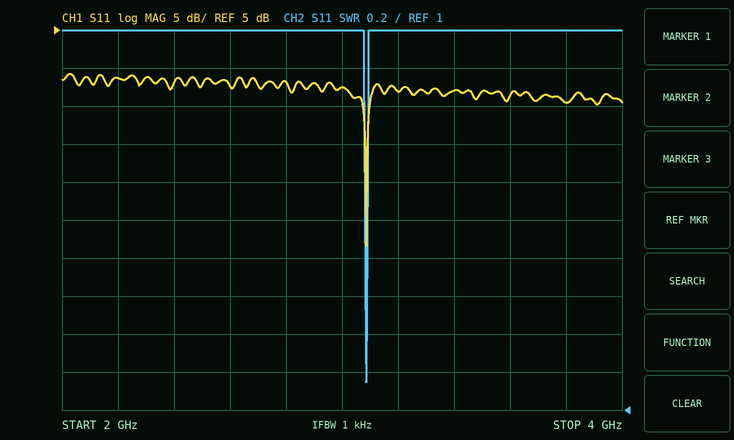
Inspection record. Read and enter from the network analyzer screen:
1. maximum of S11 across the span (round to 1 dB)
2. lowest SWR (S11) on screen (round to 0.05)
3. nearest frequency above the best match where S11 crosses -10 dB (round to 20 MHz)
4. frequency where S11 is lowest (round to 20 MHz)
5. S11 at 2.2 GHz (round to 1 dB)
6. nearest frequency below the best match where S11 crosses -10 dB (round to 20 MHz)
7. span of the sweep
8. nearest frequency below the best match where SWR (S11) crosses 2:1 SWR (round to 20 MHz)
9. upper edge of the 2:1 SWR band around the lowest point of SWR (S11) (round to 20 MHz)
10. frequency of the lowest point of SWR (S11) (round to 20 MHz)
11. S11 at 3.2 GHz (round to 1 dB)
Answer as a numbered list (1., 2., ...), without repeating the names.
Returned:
1. -1 dB
2. 1.15
3. 3.10 GHz
4. 3.08 GHz
5. -1 dB
6. 3.08 GHz
7. 2 GHz
8. 3.08 GHz
9. 3.10 GHz
10. 3.08 GHz
11. -3 dB
